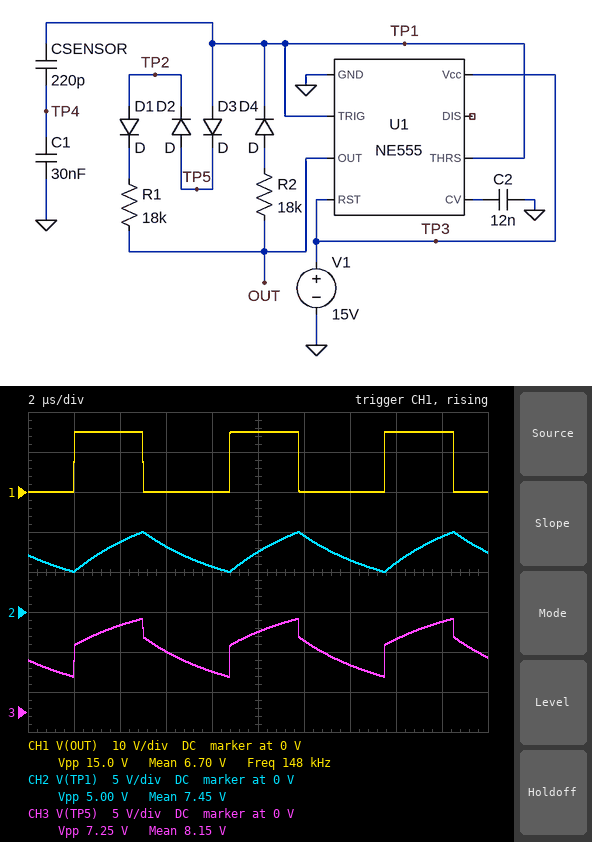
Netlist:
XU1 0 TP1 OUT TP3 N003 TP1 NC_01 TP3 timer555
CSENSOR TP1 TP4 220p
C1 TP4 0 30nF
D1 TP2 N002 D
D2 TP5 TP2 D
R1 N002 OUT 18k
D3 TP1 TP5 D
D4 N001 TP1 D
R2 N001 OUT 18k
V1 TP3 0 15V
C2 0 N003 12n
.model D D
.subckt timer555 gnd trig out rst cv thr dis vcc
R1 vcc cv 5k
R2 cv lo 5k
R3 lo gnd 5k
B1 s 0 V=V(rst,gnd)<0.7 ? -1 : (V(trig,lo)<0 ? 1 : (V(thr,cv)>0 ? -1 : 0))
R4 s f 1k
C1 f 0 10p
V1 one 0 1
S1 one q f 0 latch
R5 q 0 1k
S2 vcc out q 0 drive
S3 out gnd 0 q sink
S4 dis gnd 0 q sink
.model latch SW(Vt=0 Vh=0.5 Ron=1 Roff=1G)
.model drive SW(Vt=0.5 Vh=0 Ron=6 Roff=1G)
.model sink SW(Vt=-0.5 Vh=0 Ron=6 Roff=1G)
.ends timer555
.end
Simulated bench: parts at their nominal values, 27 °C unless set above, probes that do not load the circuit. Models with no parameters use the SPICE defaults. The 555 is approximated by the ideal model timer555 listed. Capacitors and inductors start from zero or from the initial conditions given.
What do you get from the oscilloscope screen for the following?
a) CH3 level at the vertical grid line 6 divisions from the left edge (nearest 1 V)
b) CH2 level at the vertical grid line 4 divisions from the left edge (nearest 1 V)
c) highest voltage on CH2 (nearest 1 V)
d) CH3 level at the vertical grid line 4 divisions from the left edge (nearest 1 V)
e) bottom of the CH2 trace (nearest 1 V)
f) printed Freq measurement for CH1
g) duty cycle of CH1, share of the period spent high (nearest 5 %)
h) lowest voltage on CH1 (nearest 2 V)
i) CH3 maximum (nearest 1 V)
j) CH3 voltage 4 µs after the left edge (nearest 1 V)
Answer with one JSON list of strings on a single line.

["9 V", "6 V", "10 V", "5 V", "5 V", "148 kHz", "45 %", "0 V", "12 V", "11 V"]
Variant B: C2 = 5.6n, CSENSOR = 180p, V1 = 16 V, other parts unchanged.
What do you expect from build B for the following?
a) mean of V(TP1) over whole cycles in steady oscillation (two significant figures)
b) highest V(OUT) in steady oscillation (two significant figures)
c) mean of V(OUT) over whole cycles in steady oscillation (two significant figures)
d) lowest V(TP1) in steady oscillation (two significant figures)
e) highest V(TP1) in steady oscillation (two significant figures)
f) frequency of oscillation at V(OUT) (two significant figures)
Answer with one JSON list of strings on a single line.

["7.9 V", "16 V", "7.2 V", "5.3 V", "11 V", "180 kHz"]
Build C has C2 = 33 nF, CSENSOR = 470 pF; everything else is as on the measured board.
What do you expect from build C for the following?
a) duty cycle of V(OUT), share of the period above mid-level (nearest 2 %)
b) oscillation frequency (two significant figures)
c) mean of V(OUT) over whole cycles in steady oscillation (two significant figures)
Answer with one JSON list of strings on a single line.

["42 %", "72 kHz", "6.4 V"]
